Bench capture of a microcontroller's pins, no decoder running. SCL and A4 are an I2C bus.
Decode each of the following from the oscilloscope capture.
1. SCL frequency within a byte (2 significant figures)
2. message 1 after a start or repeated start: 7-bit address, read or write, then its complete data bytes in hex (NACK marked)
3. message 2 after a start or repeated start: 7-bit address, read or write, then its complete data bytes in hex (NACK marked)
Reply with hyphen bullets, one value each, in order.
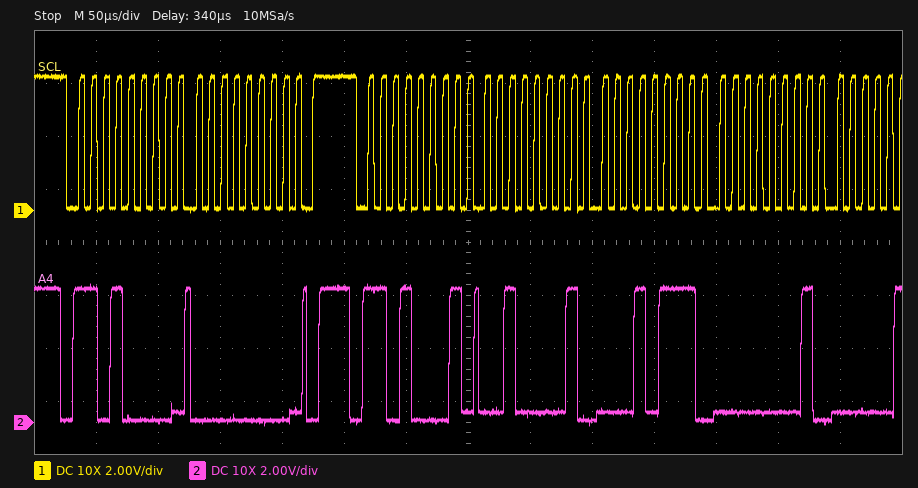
- 100 kHz
- 0x68 write: 00
- 0x68 read: 21 17 01
